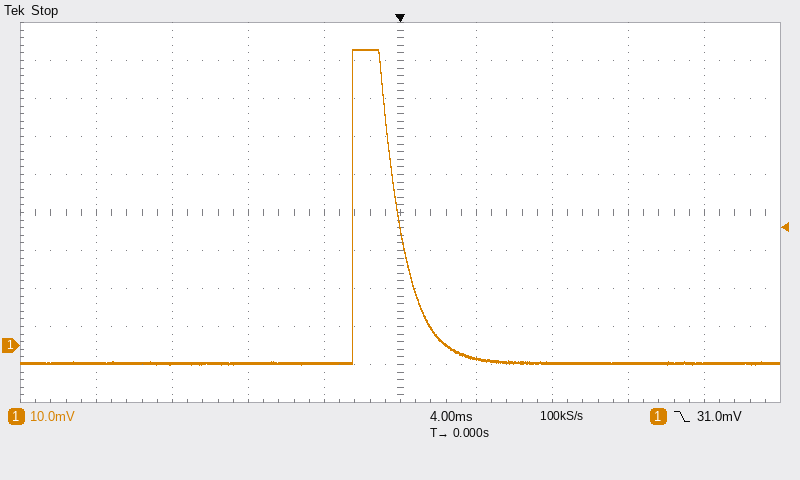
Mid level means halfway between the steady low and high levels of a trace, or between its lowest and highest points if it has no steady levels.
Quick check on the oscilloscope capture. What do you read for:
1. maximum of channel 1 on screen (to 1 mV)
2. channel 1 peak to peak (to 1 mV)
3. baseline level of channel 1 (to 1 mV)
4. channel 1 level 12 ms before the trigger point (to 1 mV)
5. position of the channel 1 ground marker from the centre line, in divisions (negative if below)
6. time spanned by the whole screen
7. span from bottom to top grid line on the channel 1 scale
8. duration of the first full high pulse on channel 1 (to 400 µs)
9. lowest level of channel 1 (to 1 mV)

78 mV
83 mV
-5 mV
-5 mV
-3.5 div
40 ms
100 mV
2.4 ms
-5 mV
